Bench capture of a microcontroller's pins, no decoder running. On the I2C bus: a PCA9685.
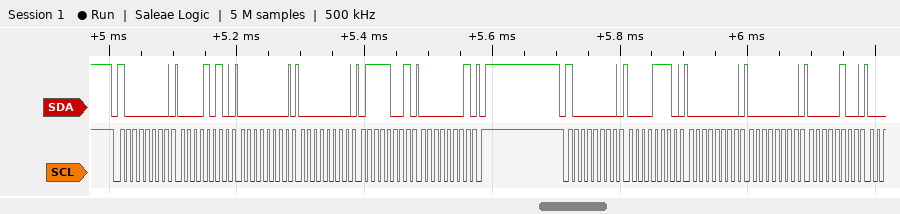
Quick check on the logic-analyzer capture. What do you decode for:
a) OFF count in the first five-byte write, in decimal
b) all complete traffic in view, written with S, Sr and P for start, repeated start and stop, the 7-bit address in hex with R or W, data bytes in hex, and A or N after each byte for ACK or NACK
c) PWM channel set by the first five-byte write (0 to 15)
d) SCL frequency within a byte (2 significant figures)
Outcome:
377
S 40W A 0A A 00 A 00 A 79 A 01 A P S 40W A 0E A 00 A 00 A 04 A
1
100 kHz
